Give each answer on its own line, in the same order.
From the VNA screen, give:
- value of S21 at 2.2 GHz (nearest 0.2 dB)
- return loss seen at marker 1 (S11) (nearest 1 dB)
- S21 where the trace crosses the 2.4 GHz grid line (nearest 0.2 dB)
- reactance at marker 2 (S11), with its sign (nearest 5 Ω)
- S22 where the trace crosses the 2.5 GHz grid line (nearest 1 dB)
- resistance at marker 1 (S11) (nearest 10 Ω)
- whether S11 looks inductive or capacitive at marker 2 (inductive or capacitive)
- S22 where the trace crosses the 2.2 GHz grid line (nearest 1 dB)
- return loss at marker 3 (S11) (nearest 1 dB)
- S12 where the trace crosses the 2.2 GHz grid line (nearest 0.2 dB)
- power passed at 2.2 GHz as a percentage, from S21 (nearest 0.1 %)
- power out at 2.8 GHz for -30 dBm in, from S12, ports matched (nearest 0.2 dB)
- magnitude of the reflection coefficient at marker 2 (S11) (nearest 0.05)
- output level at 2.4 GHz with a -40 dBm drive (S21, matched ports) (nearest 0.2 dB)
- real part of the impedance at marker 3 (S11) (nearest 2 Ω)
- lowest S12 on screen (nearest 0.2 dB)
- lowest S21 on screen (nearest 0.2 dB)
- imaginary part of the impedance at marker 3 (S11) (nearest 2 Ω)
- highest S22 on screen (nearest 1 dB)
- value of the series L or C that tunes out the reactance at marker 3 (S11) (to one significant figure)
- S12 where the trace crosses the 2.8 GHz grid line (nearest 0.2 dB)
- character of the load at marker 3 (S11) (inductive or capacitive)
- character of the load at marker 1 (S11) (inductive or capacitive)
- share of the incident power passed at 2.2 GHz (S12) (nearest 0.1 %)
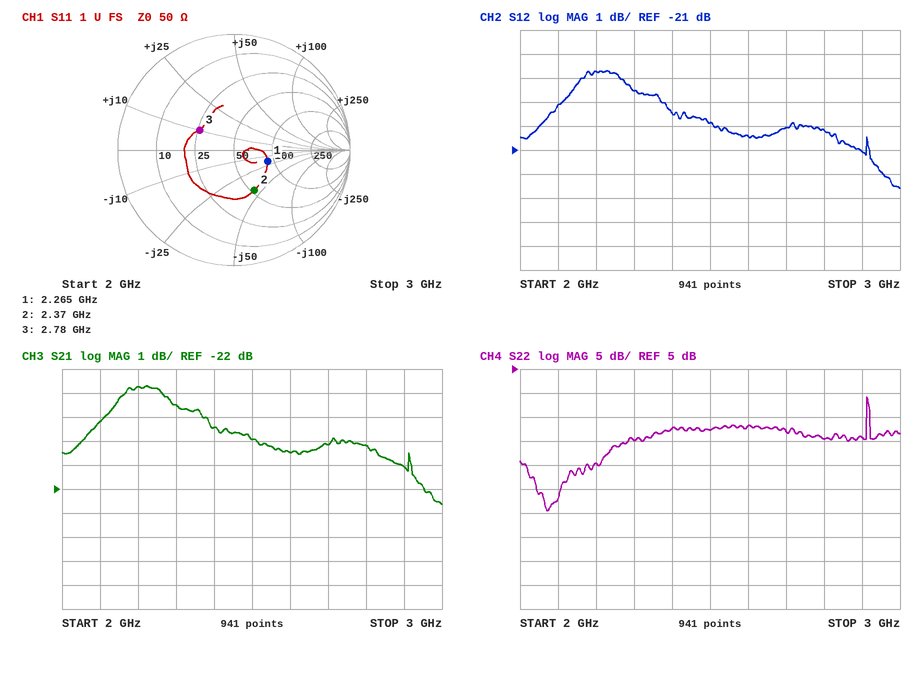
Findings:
-17.8 dB
10 dB
-19.4 dB
-45 Ω
-8 dB
90 Ω
capacitive
-15 dB
9 dB
-17.8 dB
1.7 %
-50.2 dBm
0.40
-59.4 dBm
26 Ω
-22.6 dB
-22.6 dB
+10 Ω
-1 dB
6 pF
-20.2 dB
inductive
capacitive
1.7 %
